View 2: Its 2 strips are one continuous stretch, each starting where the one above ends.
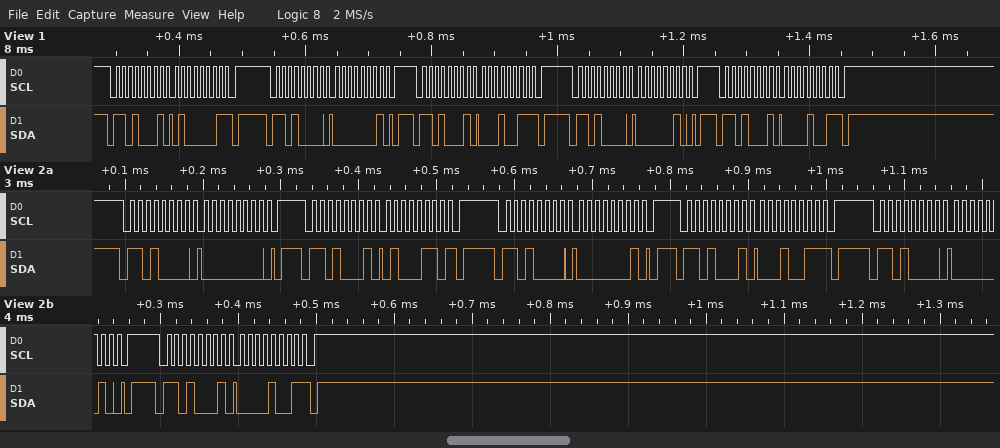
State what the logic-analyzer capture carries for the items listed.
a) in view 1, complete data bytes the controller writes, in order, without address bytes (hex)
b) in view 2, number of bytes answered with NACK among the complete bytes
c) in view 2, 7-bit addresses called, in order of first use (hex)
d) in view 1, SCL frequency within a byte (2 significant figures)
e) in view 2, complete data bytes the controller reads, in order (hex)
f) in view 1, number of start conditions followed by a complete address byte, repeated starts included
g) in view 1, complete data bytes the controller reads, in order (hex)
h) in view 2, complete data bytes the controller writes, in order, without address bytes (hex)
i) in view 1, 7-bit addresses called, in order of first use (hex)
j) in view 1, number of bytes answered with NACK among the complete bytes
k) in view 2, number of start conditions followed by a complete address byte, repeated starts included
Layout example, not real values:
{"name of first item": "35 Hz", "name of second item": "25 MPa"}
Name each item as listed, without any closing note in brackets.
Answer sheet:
{"in view 1, complete data bytes the controller writes, in order, without address bytes": "01 02", "in view 2, number of bytes answered with NACK among the complete bytes": "3", "in view 2, 7-bit addresses called, in order of first use": "0x68", "in view 1, SCL frequency within a byte": "100 kHz", "in view 2, complete data bytes the controller reads, in order": "46 13 09", "in view 1, number of start conditions followed by a complete address byte, repeated starts included": "5", "in view 1, complete data bytes the controller reads, in order": "41 13 09", "in view 2, complete data bytes the controller writes, in order, without address bytes": "00 01 02", "in view 1, 7-bit addresses called, in order of first use": "0x68", "in view 1, number of bytes answered with NACK among the complete bytes": "3", "in view 2, number of start conditions followed by a complete address byte, repeated starts included": "6"}
